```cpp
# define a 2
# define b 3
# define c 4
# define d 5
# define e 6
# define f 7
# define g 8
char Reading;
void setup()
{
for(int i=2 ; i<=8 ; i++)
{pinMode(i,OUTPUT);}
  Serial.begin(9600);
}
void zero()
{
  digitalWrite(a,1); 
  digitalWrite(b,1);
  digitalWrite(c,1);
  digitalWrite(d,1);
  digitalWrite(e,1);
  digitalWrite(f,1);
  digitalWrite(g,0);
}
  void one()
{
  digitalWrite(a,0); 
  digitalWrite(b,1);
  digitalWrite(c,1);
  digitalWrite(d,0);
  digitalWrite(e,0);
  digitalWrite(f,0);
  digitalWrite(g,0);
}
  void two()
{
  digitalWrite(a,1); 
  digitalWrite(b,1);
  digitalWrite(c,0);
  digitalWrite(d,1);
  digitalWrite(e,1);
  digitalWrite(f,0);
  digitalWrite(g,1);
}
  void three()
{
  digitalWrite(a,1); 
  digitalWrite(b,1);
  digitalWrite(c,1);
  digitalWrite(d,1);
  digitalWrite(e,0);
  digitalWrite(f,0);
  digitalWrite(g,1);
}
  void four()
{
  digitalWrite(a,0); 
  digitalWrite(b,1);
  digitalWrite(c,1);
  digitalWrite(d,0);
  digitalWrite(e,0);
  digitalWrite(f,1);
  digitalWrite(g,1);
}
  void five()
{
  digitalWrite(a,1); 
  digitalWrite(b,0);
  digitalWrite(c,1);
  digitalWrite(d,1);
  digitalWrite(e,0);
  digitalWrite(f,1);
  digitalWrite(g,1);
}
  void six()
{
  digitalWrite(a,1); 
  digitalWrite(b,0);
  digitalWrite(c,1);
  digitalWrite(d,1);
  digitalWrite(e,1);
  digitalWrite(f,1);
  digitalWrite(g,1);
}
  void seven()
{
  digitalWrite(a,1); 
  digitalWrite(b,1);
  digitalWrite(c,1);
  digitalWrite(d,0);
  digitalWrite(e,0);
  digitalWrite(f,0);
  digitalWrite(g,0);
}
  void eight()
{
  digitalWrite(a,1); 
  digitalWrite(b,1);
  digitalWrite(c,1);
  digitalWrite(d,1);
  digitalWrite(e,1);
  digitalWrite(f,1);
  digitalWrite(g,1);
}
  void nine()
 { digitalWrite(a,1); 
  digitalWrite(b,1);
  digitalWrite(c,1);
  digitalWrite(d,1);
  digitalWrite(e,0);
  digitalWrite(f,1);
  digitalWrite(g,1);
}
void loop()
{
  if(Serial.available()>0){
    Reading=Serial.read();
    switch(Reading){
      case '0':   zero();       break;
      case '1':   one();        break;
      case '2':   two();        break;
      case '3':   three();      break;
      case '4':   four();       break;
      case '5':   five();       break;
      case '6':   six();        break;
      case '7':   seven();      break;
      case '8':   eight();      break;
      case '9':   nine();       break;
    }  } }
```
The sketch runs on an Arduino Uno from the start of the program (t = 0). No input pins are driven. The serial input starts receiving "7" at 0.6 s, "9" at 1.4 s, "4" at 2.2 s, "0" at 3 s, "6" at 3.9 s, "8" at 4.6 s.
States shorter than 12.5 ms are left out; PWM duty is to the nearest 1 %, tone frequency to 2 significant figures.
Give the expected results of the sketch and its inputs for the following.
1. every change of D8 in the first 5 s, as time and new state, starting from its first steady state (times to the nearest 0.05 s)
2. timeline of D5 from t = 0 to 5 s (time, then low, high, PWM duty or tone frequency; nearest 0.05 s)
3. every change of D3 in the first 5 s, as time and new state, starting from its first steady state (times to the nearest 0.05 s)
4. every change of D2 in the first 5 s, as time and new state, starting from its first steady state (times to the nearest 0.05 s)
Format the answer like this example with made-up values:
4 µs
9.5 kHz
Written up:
0 s low; 1.4 s high; 3 s low; 3.9 s high
0 s low; 1.4 s high; 2.2 s low; 3 s high
0 s low; 0.6 s high; 3.9 s low; 4.6 s high
0 s low; 0.6 s high; 2.2 s low; 3 s high
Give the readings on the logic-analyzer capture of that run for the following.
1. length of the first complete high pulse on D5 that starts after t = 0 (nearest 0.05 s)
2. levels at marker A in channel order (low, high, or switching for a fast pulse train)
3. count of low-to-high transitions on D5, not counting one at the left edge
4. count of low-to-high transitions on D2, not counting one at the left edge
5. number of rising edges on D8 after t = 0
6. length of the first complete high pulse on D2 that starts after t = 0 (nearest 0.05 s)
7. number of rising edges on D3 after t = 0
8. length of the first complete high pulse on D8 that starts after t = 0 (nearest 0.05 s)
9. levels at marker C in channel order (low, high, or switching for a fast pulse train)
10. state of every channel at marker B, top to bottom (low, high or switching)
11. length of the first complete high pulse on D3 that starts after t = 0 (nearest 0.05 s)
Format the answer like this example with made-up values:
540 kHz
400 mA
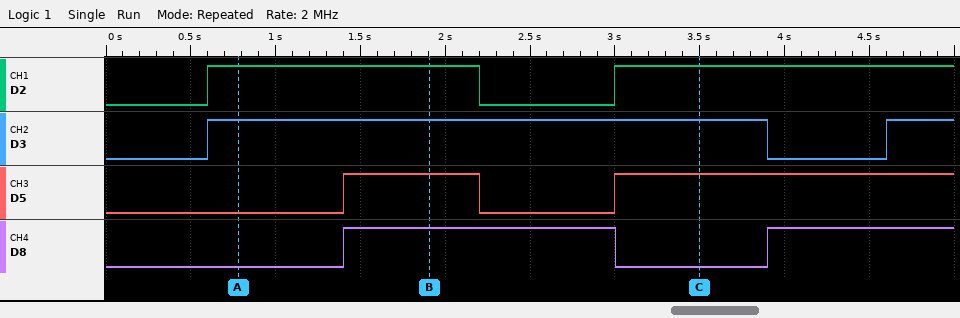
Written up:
0.80 s
D2 high, D3 high, D5 low, D8 low
2
2
2
1.60 s
2
1.60 s
D2 high, D3 high, D5 high, D8 low
D2 high, D3 high, D5 high, D8 high
3.30 s
